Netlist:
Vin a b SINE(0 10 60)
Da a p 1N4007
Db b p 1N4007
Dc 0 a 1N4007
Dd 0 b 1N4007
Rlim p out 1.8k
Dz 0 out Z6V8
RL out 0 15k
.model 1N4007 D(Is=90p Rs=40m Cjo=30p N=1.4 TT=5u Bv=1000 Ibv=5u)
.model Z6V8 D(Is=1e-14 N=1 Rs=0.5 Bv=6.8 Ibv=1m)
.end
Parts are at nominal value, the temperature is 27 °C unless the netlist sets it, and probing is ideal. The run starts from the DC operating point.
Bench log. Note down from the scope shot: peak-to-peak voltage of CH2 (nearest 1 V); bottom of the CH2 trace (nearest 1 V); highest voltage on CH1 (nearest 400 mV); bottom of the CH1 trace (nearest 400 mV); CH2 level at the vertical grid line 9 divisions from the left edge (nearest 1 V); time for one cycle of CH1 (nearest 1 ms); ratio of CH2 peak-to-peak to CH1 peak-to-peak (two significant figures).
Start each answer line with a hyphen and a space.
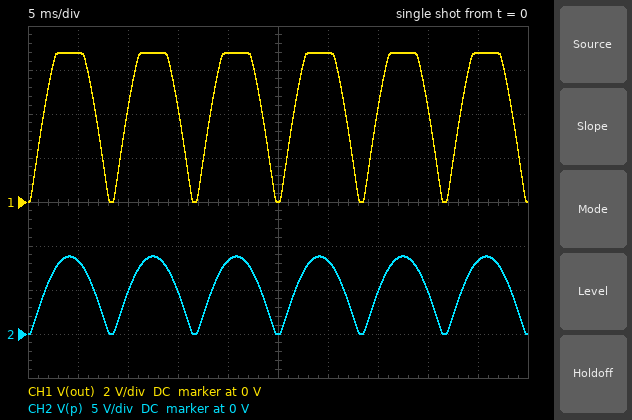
- 9 V
- 0 V
- 6.8 V
- 0 V
- 8 V
- 8 ms
- 1.3
